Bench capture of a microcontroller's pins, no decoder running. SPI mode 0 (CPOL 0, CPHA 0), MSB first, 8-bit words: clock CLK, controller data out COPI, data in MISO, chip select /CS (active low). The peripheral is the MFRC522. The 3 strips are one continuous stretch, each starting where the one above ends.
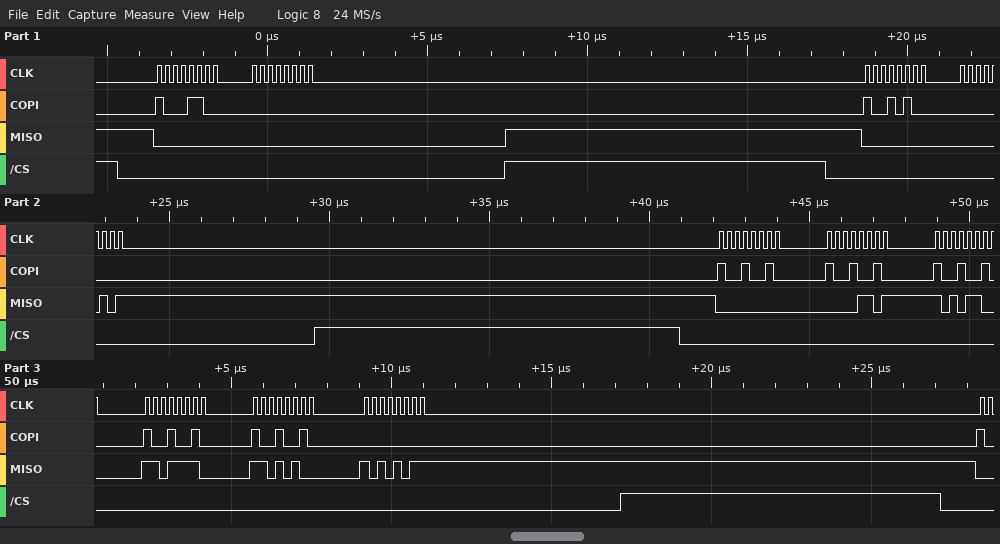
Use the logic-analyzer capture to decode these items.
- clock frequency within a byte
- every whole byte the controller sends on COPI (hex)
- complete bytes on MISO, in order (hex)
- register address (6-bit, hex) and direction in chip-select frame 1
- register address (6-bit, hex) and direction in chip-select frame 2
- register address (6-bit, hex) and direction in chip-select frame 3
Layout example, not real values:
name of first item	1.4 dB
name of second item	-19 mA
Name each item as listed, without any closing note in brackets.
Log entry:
clock frequency within a byte	4 MHz
every whole byte the controller sends on COPI	8C 00 94 00 92 92 92 92 92 00
complete bytes on MISO, in order	00 00 00 05 00 0D AC DE D4 AB
register address (6-bit, hex) and direction in chip-select frame 1	0x06 read
register address (6-bit, hex) and direction in chip-select frame 2	0x0A read
register address (6-bit, hex) and direction in chip-select frame 3	0x09 read
